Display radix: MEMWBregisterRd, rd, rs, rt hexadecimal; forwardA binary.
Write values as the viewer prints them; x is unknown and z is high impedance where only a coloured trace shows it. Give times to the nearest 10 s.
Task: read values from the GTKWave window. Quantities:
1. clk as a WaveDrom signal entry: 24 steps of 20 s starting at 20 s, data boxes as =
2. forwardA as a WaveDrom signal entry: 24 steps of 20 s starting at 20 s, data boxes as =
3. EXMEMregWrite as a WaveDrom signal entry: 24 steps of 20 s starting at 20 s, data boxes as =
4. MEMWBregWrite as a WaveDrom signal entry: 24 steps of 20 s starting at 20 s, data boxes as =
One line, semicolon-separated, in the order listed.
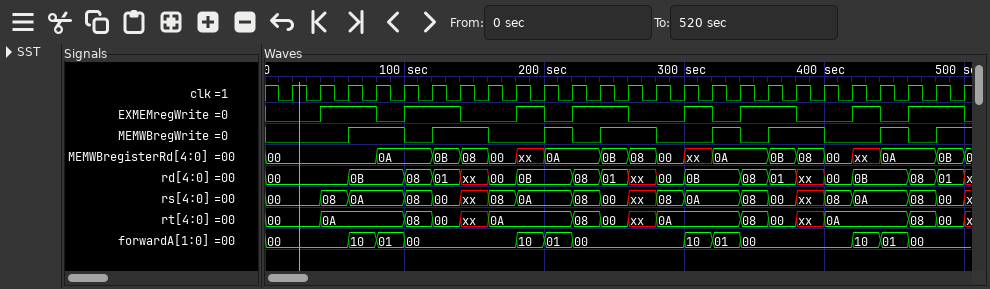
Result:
{name: 'clk', wave: 'p.......................'}; {name: 'forwardA', wave: '=.===...===...===...===.', data: '00 10 01 00 10 01 00 10 01 00 10 01 00'}; {name: 'EXMEMregWrite', wave: '01.01.0.101.0.101.0.101.'}; {name: 'MEMWBregWrite', wave: '0.1.01.0.101.0.101.0.101'}
